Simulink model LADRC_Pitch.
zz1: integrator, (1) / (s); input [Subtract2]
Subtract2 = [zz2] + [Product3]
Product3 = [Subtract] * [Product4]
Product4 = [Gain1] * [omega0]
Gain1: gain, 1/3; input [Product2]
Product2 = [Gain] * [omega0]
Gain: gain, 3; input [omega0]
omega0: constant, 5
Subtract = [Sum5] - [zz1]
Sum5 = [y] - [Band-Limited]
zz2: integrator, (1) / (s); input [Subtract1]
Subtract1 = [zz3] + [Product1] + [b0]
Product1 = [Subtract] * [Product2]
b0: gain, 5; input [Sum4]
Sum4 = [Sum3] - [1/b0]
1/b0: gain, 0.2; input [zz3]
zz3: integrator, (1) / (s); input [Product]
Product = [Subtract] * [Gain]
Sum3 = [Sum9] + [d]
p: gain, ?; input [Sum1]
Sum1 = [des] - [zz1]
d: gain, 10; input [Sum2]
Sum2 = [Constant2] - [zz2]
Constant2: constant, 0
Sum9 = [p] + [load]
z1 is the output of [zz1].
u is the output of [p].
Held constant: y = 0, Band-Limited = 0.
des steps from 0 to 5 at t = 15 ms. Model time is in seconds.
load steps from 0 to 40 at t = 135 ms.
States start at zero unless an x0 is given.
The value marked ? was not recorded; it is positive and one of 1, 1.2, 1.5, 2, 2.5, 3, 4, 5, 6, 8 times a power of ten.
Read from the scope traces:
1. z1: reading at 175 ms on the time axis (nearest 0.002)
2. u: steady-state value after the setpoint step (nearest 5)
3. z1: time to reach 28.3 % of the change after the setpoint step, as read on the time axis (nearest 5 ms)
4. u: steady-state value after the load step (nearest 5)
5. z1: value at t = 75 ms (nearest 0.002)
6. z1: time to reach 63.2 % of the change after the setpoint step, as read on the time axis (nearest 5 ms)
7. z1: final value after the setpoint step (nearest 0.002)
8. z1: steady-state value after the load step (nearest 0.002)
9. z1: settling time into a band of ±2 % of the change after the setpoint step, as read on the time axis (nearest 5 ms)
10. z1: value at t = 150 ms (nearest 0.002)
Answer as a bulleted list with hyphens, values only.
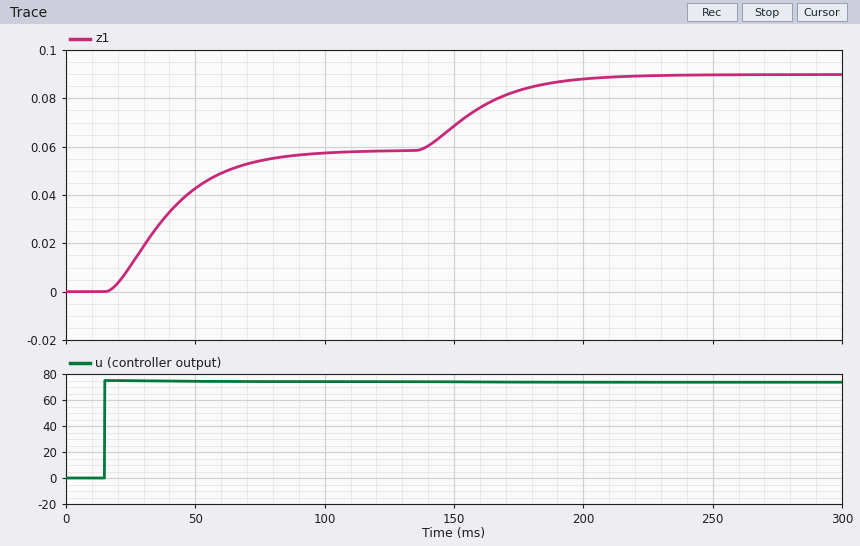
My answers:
- 0.084
- 75
- 30 ms
- 75
- 0.054
- 45 ms
- 0.058
- 0.090
- 100 ms
- 0.068
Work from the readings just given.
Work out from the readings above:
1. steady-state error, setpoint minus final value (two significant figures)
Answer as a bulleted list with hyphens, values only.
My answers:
- 4.9
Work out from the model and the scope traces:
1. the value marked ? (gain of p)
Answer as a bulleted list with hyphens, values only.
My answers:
- 15
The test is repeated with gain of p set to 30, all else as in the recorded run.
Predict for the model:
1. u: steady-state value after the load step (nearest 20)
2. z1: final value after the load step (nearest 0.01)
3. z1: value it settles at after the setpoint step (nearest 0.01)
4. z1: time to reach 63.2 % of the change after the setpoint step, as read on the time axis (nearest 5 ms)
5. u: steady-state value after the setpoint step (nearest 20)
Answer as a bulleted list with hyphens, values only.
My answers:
- 140
- 0.15
- 0.12
- 45 ms
- 140
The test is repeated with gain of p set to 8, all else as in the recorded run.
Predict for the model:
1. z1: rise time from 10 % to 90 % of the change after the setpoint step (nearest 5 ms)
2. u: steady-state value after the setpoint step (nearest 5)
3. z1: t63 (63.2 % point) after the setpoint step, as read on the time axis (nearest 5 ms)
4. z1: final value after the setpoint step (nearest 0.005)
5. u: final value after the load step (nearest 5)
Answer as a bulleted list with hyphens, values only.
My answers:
- 50 ms
- 40
- 45 ms
- 0.030
- 40
